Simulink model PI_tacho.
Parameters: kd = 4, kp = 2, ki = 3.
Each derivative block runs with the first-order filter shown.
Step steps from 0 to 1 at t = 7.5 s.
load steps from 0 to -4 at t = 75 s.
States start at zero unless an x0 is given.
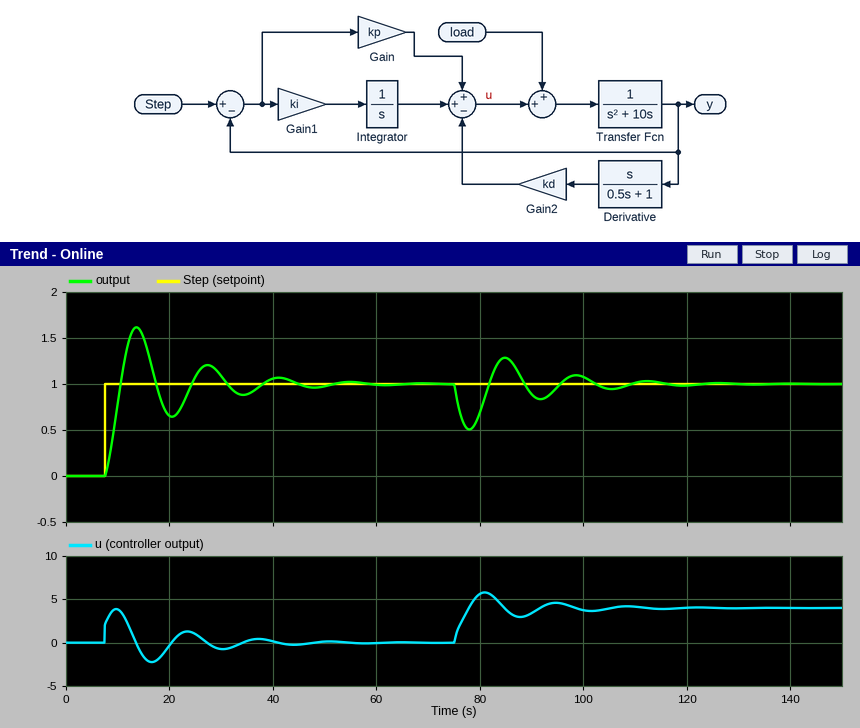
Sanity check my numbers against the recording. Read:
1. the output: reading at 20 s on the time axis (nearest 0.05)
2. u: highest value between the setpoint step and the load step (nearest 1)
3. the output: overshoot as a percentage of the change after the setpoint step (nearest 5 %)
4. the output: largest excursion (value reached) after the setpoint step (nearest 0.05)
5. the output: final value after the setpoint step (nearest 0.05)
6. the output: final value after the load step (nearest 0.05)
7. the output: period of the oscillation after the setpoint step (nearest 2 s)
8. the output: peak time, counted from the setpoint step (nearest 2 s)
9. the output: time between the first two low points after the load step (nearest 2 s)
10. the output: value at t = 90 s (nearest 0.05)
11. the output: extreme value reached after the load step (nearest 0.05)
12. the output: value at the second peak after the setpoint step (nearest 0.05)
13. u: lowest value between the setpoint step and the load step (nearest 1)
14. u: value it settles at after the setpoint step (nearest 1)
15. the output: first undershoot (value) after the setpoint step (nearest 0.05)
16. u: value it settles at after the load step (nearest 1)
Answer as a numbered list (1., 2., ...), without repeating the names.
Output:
1. 0.65
2. 4
3. 60 %
4. 1.60
5. 1.00
6. 1.00
7. 14 s
8. 6 s
9. 14 s
10. 0.90
11. 0.50
12. 1.20
13. -2
14. 0
15. 0.65
16. 4
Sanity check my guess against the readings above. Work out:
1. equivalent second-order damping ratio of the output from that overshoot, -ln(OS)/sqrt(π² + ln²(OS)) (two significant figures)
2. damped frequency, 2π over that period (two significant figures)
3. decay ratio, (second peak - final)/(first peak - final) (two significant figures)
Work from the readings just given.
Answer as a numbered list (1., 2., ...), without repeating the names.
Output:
1. 0.16
2. 0.45 rad/s
3. 0.33
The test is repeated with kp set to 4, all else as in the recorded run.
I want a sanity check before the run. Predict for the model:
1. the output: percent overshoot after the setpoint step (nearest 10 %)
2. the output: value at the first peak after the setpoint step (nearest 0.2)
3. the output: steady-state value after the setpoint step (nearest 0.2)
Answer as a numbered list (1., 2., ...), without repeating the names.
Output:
1. 40 %
2. 1.4
3. 1.0
